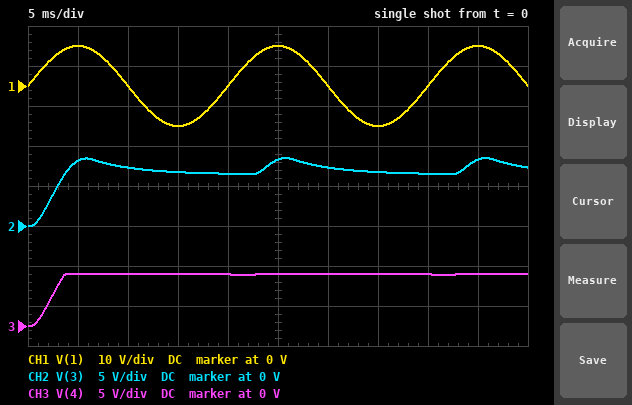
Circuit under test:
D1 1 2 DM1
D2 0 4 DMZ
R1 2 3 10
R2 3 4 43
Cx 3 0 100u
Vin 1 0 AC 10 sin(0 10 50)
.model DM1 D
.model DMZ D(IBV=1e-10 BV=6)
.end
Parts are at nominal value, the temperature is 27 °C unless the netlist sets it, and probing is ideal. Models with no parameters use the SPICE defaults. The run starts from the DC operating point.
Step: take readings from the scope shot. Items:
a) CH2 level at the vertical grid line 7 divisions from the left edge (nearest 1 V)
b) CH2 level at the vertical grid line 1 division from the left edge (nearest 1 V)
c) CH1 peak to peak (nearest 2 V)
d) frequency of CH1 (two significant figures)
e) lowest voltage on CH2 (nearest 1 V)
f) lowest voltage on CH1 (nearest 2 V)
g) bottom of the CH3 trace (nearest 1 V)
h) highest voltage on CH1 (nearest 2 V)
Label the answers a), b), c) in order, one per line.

a) 7 V
b) 8 V
c) 20 V
d) 50 Hz
e) 0 V
f) -10 V
g) 0 V
h) 10 V
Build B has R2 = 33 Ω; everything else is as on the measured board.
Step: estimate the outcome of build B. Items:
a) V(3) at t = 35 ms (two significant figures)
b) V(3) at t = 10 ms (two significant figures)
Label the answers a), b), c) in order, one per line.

a) 6.6 V
b) 7.1 V
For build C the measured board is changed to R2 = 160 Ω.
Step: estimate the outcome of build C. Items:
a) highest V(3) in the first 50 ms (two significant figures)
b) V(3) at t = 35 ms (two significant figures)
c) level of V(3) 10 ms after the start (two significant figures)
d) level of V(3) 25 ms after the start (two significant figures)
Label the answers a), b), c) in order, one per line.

a) 8.8 V
b) 7.8 V
c) 8.2 V
d) 8.6 V
